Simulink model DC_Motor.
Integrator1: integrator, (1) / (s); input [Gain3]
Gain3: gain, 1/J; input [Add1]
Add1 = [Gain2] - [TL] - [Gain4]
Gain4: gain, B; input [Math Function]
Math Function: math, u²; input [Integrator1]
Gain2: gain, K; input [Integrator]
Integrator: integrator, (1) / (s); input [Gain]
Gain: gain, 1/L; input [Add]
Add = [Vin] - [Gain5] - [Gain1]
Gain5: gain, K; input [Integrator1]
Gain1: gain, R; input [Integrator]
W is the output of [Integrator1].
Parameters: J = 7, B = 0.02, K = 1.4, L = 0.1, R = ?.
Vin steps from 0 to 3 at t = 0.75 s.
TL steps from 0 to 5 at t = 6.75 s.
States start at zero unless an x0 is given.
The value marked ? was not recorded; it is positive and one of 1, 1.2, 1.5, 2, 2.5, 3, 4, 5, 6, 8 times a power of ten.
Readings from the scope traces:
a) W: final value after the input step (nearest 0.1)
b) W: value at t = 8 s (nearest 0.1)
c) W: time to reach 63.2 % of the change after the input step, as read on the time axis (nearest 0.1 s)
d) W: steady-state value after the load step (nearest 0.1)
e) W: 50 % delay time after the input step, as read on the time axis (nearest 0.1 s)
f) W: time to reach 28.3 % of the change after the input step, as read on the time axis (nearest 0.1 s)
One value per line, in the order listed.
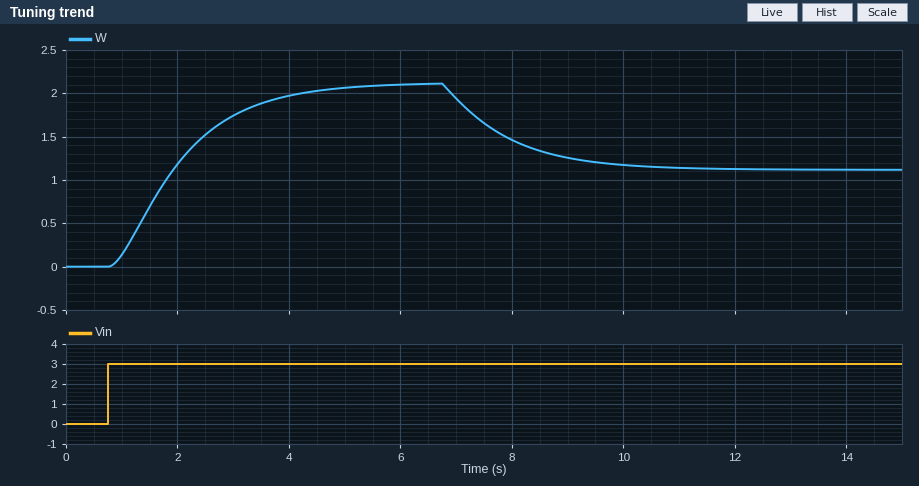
2.1
1.5
2.2 s
1.1
1.9 s
1.4 s
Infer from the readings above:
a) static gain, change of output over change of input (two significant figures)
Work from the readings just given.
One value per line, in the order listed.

0.70
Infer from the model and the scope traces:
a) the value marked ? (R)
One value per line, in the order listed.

0.4
